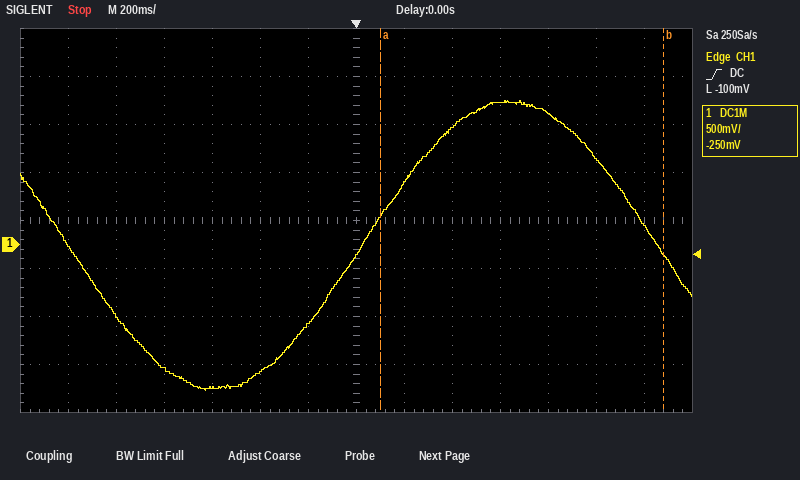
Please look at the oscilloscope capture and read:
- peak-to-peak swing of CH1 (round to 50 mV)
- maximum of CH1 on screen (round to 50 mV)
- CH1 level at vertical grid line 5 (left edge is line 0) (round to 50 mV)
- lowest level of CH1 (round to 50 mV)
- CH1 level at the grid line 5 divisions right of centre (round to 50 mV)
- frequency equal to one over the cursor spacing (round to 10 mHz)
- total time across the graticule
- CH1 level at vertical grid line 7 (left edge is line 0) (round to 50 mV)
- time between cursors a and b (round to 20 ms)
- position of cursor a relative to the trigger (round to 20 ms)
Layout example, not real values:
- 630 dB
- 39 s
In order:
- 3.00 V
- 1.50 V
- -1.30 V
- -1.50 V
- 900 mV
- 850 mHz
- 2.8 s
- -100 mV
- 1.18 s
- +100 ms
